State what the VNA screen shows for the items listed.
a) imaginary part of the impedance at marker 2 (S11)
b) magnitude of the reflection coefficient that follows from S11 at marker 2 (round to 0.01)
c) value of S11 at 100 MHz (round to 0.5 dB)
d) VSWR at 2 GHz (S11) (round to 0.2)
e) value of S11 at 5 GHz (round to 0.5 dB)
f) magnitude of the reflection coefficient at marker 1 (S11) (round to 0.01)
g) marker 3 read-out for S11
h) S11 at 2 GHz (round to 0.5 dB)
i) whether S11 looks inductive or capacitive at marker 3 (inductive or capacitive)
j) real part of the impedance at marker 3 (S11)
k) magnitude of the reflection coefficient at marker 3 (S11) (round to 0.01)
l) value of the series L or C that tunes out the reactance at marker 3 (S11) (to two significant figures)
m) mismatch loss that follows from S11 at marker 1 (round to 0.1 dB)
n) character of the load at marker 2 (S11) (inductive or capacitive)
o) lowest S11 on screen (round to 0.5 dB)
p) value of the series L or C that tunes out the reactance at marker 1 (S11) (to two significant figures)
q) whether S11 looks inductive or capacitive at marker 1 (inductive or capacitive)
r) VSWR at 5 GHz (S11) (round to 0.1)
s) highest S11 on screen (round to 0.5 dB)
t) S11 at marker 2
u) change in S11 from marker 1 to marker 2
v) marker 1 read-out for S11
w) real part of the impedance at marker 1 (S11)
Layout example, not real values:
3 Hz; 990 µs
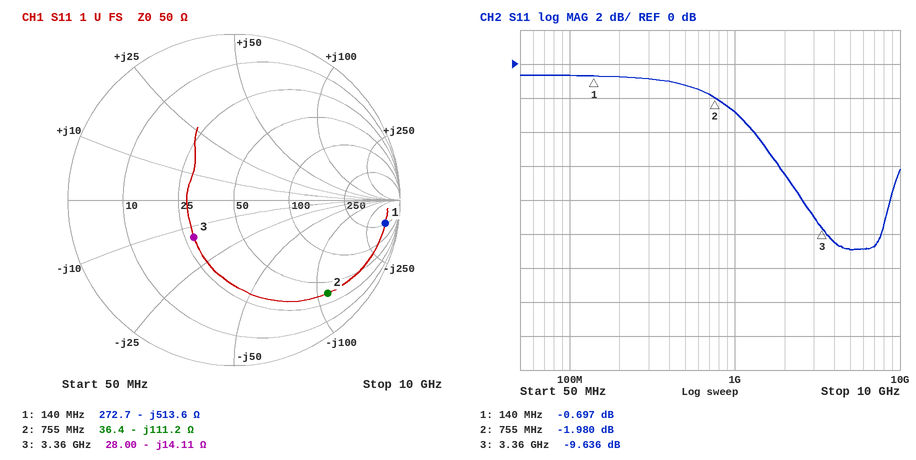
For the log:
-111.2 Ω; 0.80; -0.5 dB; 2.8; -11.0 dB; 0.92; -9.636 dB; -6.5 dB; capacitive; 28.00 Ω; 0.33; 670 pH; 8.3 dB; capacitive; -11.0 dB; 580 nH; capacitive; 1.8; -0.5 dB; -1.980 dB; -1.283 dB; -0.697 dB; 272.7 Ω
